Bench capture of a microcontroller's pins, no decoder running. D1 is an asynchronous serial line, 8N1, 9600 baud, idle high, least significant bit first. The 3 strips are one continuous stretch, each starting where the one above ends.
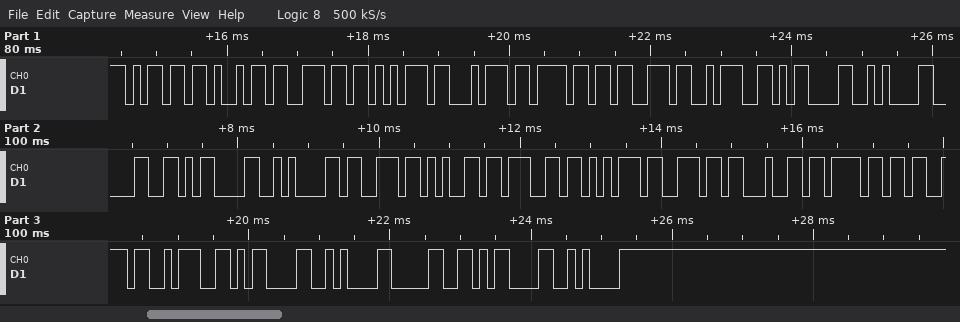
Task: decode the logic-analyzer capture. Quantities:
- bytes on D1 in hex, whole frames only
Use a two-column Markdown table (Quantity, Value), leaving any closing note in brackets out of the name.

| Quantity | Value |
|---|---|
| bytes on D1 in hex, whole frames only | 6D 69 6E 75 74 6F 73 3A 0D 0A 30 0D 0A 73 65 67 75 6E 64 6F 73 3A 0D 0A 30 0D 0A |
